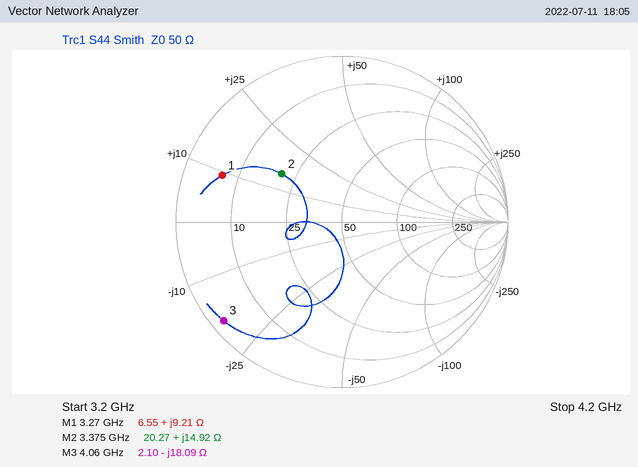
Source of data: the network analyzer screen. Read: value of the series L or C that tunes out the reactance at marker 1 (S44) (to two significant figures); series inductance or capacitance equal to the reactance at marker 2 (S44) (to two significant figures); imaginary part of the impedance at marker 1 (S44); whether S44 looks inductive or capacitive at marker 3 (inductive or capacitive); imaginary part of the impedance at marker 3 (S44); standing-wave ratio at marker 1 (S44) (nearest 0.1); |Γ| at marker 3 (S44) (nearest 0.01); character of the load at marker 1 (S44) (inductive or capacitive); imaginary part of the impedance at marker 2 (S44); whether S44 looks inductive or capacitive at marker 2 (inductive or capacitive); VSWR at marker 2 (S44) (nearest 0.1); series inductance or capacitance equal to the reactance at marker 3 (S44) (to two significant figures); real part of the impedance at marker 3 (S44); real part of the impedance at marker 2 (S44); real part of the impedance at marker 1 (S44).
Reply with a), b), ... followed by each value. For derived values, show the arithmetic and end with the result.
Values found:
a) C = 1/(2π × 3.27 GHz × 9.21 Ω) ≈ 5.3 pF
b) L = 14.92 Ω/(2π × 3.375 GHz) ≈ 704 pH, so 700 pH to two significant figures
c) +9.21 Ω
d) capacitive
e) -18.09 Ω
f) 7.9
g) 0.93
h) inductive
i) +14.92 Ω
j) inductive
k) 2.7
l) C = 1/(2π × 4.06 GHz × 18.09 Ω) ≈ 2.2 pF
m) 2.10 Ω
n) 20.27 Ω
o) 6.55 Ω
